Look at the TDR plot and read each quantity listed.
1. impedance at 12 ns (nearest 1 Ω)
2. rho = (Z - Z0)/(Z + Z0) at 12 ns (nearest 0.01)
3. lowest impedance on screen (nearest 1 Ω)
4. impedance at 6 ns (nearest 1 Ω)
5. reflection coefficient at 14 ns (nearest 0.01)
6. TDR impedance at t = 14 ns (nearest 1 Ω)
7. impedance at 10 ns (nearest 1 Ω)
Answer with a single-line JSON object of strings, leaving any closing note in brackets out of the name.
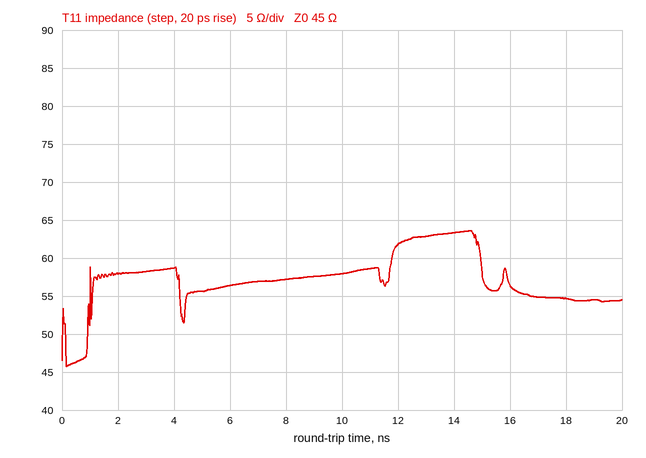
{"impedance at 12 ns": "62 Ω", "rho = (Z - Z0)/(Z + Z0) at 12 ns": "+0.16", "lowest impedance on screen": "46 Ω", "impedance at 6 ns": "56 Ω", "reflection coefficient at 14 ns": "+0.17", "TDR impedance at t = 14 ns": "63 Ω", "impedance at 10 ns": "58 Ω"}
